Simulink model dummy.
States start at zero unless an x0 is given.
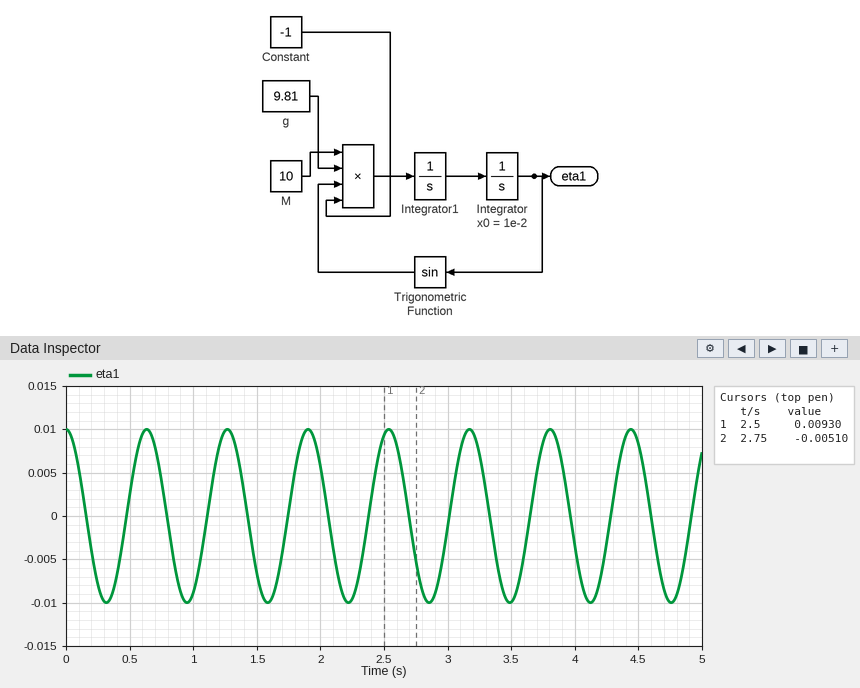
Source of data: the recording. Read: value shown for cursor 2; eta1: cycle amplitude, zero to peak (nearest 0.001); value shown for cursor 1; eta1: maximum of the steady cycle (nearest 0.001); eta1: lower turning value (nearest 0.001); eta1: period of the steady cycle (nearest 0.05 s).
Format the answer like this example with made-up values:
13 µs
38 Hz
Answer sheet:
-0.00510
0.010
0.00930
0.010
-0.010
0.65 s
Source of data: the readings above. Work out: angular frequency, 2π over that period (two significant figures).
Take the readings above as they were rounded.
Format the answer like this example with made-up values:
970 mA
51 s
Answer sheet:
9.7 rad/s
